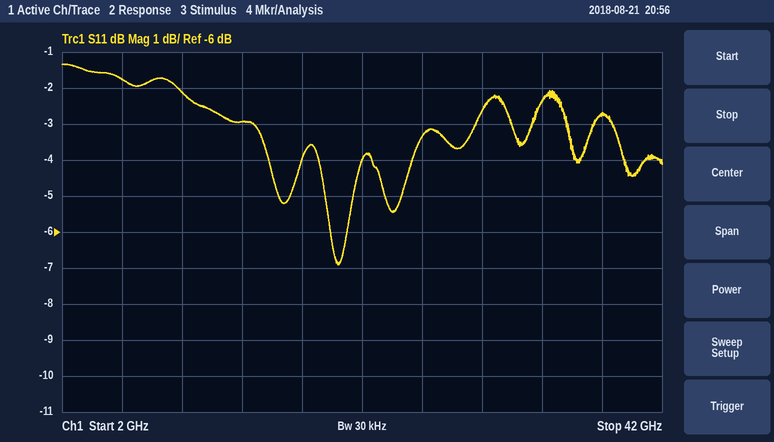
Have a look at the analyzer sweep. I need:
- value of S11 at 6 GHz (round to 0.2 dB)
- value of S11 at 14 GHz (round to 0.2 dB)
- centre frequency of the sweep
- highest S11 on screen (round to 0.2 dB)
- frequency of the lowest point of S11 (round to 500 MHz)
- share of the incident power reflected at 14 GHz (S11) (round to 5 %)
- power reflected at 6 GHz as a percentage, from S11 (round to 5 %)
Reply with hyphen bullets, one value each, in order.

- -1.8 dB
- -3.0 dB
- 22 GHz
- -1.4 dB
- 20.5 GHz
- 50 %
- 65 %
